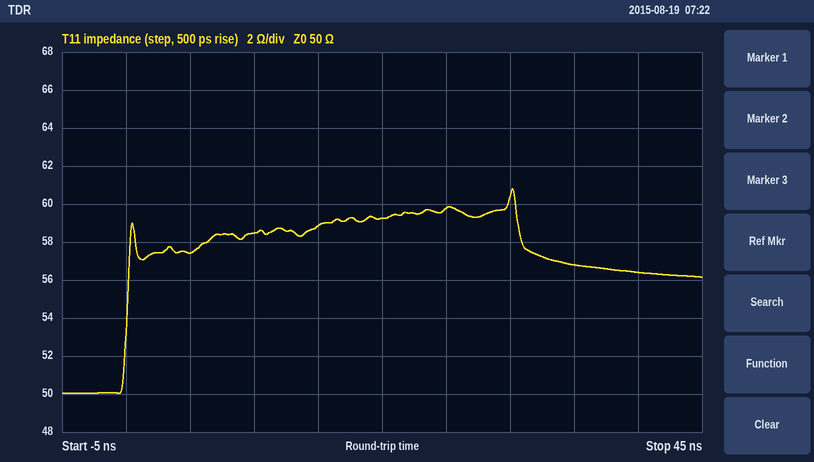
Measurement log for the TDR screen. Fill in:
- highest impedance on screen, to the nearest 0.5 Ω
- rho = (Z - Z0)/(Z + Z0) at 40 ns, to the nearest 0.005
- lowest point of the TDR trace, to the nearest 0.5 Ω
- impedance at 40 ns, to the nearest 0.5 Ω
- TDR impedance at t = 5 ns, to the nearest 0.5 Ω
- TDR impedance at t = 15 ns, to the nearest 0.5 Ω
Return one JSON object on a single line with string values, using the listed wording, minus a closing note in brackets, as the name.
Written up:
{"highest impedance on screen, to the nearest 0.5 Ω": "61.0 Ω", "rho = (Z - Z0)/(Z + Z0) at 40 ns, to the nearest 0.005": "+0.060", "lowest point of the TDR trace, to the nearest 0.5 Ω": "50.0 Ω", "impedance at 40 ns, to the nearest 0.5 Ω": "56.5 Ω", "TDR impedance at t = 5 ns, to the nearest 0.5 Ω": "57.5 Ω", "TDR impedance at t = 15 ns, to the nearest 0.5 Ω": "59.0 Ω"}
